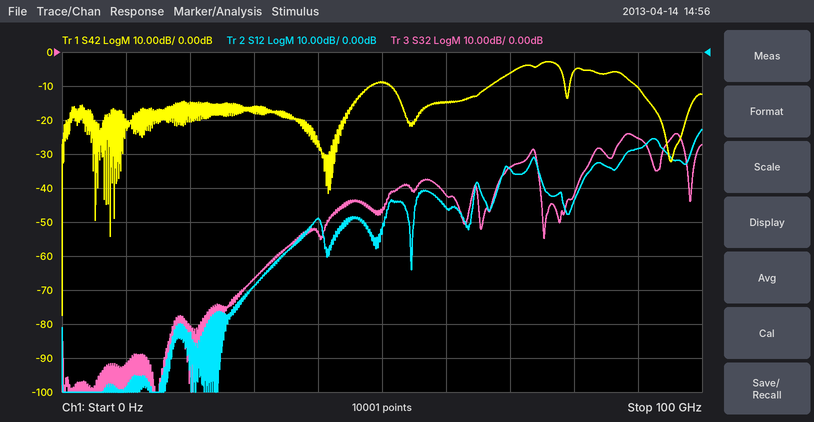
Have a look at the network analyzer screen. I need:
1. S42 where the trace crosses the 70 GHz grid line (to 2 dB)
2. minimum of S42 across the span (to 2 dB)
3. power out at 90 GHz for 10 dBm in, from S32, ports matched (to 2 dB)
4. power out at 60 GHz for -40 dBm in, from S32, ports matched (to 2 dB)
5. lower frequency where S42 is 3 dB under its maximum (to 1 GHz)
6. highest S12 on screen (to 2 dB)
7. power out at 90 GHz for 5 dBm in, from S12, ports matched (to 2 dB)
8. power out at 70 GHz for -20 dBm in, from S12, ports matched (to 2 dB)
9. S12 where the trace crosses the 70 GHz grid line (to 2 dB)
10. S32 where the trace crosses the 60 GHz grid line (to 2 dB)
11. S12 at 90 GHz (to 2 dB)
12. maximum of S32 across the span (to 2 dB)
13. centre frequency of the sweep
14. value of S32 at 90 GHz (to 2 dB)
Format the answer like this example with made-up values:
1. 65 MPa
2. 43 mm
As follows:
1. -6 dB
2. -78 dB
3. -16 dBm
4. -82 dBm
5. 70 GHz
6. -22 dB
7. -24 dBm
8. -54 dBm
9. -34 dB
10. -42 dB
11. -28 dB
12. -24 dB
13. 50 GHz
14. -26 dB
